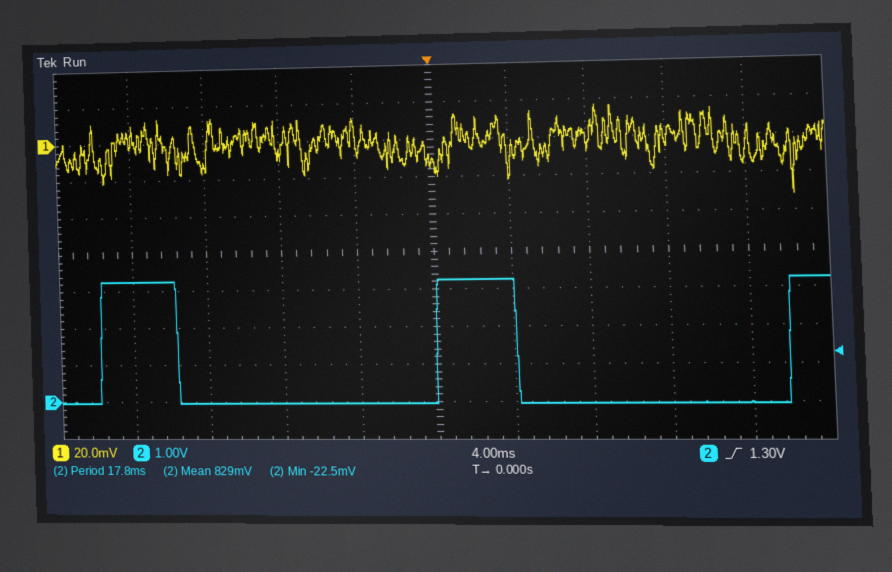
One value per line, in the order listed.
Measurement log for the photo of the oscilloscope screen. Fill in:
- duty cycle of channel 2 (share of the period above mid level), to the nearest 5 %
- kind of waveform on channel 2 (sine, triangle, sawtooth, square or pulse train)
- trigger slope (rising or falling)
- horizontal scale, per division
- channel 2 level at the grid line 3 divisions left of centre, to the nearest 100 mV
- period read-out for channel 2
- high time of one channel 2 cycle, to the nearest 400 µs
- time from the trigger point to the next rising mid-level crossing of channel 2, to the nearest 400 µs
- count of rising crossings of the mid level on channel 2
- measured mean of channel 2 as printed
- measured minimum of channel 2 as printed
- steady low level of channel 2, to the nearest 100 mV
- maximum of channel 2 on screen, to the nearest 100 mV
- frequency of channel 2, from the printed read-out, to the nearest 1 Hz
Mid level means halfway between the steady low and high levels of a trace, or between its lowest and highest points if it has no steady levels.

25 %
pulse train
rising
4 ms
0.0 V
17.8 ms
4.0 ms
18.0 ms
3
829 mV
-22.5 mV
0.0 V
3.3 V
56 Hz
